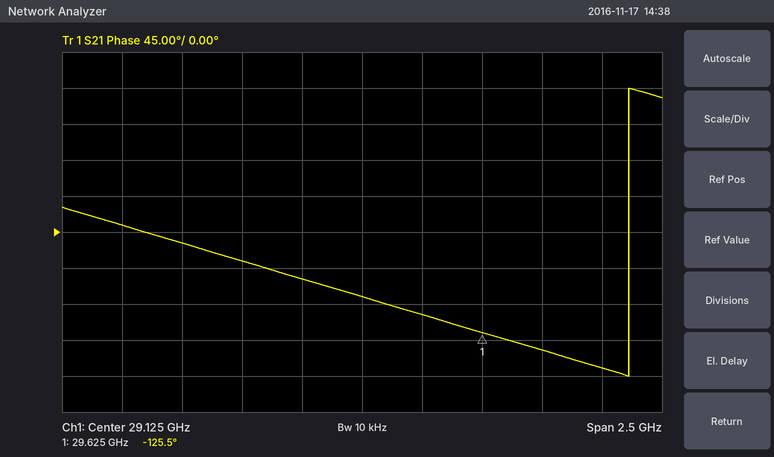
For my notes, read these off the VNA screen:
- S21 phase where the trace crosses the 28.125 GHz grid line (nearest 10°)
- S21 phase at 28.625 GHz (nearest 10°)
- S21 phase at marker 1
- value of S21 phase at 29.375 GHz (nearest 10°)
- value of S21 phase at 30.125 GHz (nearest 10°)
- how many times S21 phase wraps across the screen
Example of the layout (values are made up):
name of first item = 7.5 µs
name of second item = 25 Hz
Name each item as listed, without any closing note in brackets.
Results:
S21 phase where the trace crosses the 28.125 GHz grid line = 10°
S21 phase at 28.625 GHz = -40°
S21 phase at marker 1 = -125.5°
value of S21 phase at 29.375 GHz = -100°
value of S21 phase at 30.125 GHz = -170°
how many times S21 phase wraps across the screen = 1
